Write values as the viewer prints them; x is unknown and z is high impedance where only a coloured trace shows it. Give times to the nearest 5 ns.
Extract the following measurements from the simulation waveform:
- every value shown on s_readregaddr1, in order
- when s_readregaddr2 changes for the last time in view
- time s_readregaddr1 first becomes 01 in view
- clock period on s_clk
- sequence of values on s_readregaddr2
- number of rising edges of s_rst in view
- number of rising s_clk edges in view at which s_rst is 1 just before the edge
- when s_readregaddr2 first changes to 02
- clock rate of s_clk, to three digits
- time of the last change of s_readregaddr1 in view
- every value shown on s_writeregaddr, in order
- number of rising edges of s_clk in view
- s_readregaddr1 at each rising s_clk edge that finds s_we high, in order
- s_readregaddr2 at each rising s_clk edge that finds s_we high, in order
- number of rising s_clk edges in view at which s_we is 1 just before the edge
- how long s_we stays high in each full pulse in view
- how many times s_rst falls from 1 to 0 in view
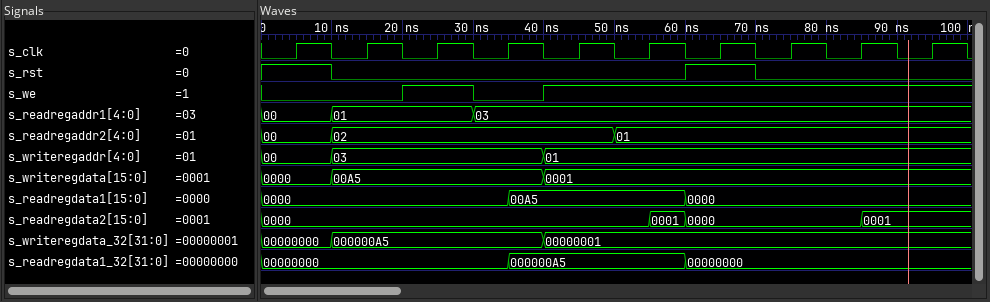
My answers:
00, 01, 03
50 ns
10 ns
10 ns
00, 02, 01
1
2
10 ns
100 MHz
30 ns
00, 03, 01
10
01, 03, 03, 03, 03, 03, 03
02, 02, 01, 01, 01, 01, 01
7
10 ns
2
